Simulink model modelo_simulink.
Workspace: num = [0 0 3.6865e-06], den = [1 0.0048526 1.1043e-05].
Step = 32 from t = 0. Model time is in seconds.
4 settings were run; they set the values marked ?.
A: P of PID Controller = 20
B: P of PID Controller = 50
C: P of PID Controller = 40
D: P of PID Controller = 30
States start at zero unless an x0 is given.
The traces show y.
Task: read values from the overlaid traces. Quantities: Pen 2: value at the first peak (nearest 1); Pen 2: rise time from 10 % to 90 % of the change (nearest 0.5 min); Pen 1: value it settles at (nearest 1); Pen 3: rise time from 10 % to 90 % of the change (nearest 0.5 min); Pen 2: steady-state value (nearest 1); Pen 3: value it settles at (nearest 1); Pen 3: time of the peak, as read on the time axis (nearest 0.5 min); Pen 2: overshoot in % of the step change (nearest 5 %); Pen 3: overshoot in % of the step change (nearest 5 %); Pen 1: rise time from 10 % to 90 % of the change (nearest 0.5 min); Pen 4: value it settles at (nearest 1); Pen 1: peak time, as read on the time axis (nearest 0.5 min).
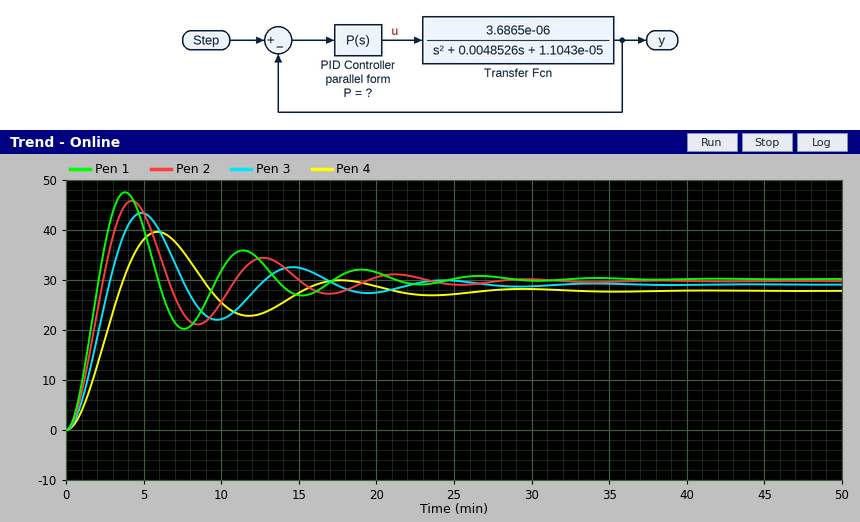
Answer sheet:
46
1.5 min
30
2.0 min
30
29
5.0 min
55 %
50 %
1.5 min
28
4.0 min
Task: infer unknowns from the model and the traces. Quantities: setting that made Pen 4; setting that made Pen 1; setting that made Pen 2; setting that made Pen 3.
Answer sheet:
A
B
C
D
